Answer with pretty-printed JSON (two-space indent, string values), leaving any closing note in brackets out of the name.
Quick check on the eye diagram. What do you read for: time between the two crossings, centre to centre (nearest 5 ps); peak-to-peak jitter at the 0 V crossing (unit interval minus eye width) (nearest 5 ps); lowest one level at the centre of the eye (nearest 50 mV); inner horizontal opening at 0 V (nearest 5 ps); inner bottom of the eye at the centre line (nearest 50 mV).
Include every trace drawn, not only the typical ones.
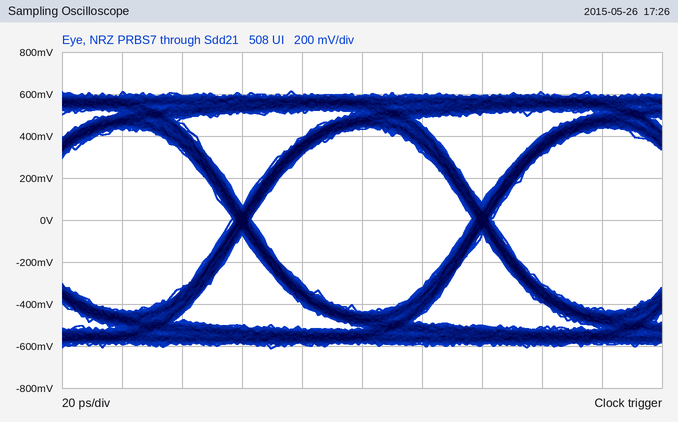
{
  "time between the two crossings, centre to centre": "80 ps",
  "peak-to-peak jitter at the 0 V crossing (unit interval minus eye width)": "5 ps",
  "lowest one level at the centre of the eye": "450 mV",
  "inner horizontal opening at 0 V": "75 ps",
  "inner bottom of the eye at the centre line": "-450 mV"
}
